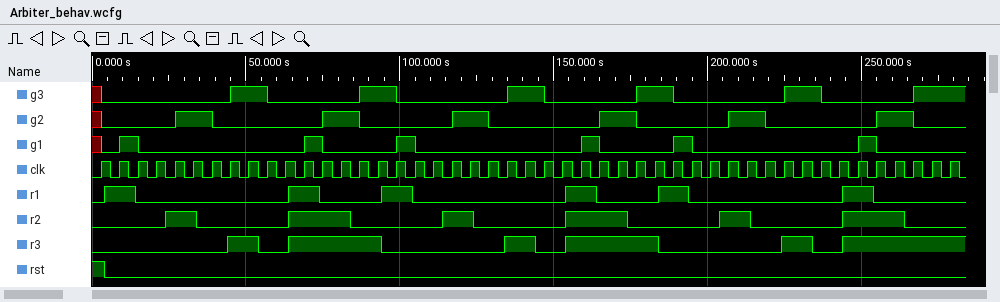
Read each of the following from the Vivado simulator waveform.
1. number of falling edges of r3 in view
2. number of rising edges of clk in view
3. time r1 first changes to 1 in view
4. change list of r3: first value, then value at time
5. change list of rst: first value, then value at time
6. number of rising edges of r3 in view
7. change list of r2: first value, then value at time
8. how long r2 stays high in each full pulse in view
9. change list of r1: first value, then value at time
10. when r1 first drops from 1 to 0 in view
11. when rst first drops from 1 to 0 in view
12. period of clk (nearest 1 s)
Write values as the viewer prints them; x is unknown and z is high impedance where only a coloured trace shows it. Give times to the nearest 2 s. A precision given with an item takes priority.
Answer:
5
47
4 s
0, 1 at 44 s, 0 at 54 s, 1 at 64 s, 0 at 94 s, 1 at 134 s, 0 at 144 s, 1 at 154 s, 0 at 184 s, 1 at 224 s, 0 at 234 s, 1 at 244 s
1, 0 at 4 s
6
0, 1 at 24 s, 0 at 34 s, 1 at 64 s, 0 at 84 s, 1 at 114 s, 0 at 124 s, 1 at 154 s, 0 at 174 s, 1 at 204 s, 0 at 214 s, 1 at 244 s, 0 at 264 s
10 s, 20 s, 10 s, 20 s, 10 s, 20 s
0, 1 at 4 s, 0 at 14 s, 1 at 64 s, 0 at 74 s, 1 at 94 s, 0 at 104 s, 1 at 154 s, 0 at 164 s, 1 at 184 s, 0 at 194 s, 1 at 244 s, 0 at 254 s
14 s
4 s
6 s
